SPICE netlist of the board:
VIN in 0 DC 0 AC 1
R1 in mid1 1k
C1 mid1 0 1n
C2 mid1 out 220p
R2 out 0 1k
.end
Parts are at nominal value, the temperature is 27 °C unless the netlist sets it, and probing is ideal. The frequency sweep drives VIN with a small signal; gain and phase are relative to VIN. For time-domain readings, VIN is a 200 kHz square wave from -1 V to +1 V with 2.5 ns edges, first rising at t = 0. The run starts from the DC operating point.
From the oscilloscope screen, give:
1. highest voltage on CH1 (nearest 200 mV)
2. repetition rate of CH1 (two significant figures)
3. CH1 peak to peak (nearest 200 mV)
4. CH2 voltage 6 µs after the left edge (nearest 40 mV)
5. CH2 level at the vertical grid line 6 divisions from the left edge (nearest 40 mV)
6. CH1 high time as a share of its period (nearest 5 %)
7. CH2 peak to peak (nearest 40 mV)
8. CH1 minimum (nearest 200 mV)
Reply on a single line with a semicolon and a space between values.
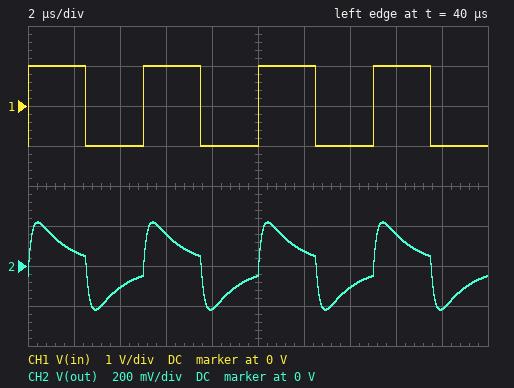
1.0 V; 200 kHz; 2.0 V; 160 mV; 80 mV; 50 %; 440 mV; -1.0 V
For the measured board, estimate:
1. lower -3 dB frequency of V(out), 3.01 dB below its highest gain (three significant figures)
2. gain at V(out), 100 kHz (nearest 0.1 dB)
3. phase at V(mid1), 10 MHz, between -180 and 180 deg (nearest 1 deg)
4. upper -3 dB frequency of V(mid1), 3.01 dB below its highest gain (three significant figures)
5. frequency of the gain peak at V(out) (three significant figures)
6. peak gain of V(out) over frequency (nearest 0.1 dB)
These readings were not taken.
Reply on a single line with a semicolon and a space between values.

101 kHz; -19.4 dB; -88 deg; 127 kHz; 339 kHz; -16.3 dB
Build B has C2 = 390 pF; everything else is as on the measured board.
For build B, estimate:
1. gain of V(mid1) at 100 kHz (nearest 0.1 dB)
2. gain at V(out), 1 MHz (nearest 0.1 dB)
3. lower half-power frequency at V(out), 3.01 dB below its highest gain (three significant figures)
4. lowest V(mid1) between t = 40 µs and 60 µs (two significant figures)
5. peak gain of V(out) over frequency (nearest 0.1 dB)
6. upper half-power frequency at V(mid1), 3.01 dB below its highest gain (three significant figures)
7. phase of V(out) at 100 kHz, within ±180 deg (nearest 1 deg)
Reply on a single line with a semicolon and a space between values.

-2.7 dB; -17.4 dB; 80.5 kHz; -710 mV; -13.2 dB; 108 kHz; 37 deg
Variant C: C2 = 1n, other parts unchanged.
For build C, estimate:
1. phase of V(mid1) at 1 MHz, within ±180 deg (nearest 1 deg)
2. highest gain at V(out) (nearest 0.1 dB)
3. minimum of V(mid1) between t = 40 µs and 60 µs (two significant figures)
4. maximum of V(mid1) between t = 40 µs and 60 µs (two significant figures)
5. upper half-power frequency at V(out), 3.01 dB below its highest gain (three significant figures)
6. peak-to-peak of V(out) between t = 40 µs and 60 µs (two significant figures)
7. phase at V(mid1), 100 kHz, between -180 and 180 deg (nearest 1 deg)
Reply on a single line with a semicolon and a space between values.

-73 deg; -9.5 dB; -600 mV; 600 mV; 526 kHz; 750 mV; -40 deg
